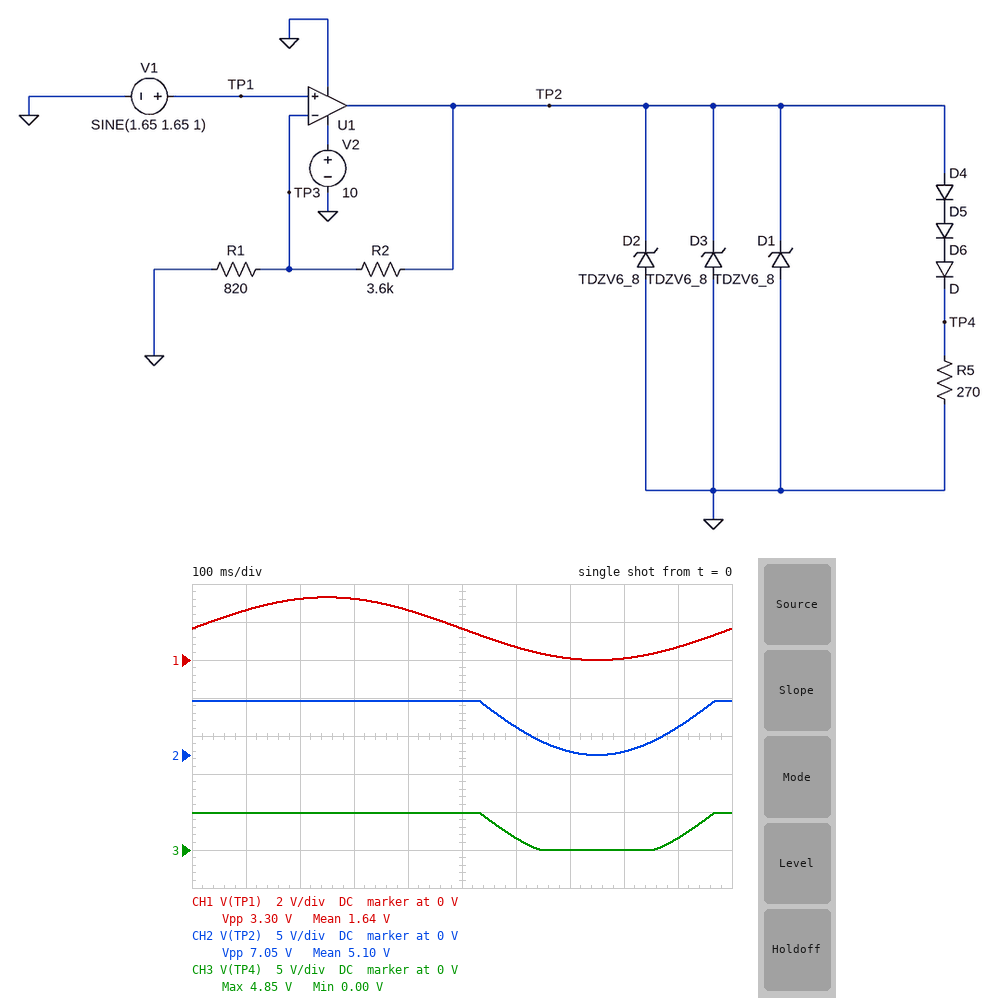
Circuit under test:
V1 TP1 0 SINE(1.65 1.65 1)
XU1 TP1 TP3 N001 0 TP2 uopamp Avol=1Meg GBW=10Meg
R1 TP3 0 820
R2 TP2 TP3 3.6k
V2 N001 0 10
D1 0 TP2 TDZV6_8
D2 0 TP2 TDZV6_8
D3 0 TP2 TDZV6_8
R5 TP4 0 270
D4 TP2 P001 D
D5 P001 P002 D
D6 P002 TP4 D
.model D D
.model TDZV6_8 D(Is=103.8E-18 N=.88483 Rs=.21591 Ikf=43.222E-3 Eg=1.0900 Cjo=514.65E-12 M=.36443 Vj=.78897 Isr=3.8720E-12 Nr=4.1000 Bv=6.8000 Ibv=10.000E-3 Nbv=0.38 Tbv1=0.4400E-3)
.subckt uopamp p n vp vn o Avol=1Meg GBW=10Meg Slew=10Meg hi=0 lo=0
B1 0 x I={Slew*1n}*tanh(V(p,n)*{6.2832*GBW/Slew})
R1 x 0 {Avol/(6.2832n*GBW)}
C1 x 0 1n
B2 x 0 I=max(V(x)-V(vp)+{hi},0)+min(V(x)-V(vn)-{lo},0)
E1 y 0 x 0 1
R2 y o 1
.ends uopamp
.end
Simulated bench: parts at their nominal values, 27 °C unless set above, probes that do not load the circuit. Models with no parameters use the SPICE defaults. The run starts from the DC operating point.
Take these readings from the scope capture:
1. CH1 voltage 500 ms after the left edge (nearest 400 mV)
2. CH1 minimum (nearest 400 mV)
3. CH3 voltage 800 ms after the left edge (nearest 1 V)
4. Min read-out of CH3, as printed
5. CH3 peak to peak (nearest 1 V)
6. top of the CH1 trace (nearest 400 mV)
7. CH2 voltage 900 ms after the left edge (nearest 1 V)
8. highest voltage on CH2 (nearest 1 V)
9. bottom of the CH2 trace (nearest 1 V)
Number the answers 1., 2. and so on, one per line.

1. 1.6 V
2. 0 V
3. 0 V
4. 0.00 V
5. 5 V
6. 3.2 V
7. 4 V
8. 7 V
9. 0 V
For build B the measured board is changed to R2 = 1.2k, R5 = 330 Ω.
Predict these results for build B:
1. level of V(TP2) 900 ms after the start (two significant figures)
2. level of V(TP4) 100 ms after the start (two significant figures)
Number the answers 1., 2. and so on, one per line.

1. 1.7 V
2. 4.3 V
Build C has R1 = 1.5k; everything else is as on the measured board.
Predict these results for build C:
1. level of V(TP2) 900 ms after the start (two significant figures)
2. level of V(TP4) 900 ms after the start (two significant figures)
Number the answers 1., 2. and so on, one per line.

1. 2.3 V
2. 330 mV
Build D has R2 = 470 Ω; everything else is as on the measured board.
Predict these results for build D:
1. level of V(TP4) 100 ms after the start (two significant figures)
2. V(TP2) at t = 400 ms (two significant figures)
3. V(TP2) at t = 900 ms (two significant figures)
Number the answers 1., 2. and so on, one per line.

1. 2.0 V
2. 4.1 V
3. 1.1 V
